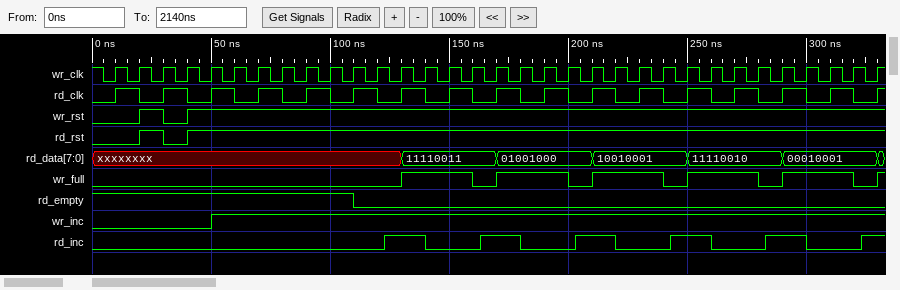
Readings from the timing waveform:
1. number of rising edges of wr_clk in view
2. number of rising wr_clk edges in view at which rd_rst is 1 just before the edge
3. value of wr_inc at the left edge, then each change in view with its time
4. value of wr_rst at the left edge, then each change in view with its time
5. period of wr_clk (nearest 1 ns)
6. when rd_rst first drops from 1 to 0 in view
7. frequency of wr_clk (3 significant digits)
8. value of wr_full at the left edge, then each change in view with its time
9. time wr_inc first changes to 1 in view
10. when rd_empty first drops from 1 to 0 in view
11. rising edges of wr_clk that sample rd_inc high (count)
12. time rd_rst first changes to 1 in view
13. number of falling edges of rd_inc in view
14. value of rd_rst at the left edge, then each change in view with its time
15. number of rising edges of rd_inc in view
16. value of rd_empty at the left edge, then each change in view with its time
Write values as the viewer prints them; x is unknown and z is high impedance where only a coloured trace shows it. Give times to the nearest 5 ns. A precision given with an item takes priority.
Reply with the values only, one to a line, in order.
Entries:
33
30
0, 1 at 50 ns
0, 1 at 20 ns, 0 at 30 ns, 1 at 40 ns
10 ns
30 ns
100 MHz
0, 1 at 130 ns, 0 at 160 ns, 1 at 170 ns, 0 at 200 ns, 1 at 210 ns, 0 at 240 ns, 1 at 250 ns, 0 at 280 ns, 1 at 290 ns, 0 at 320 ns, 1 at 330 ns
50 ns
110 ns
11
20 ns
5
0, 1 at 20 ns, 0 at 30 ns, 1 at 40 ns
6
1, 0 at 110 ns
